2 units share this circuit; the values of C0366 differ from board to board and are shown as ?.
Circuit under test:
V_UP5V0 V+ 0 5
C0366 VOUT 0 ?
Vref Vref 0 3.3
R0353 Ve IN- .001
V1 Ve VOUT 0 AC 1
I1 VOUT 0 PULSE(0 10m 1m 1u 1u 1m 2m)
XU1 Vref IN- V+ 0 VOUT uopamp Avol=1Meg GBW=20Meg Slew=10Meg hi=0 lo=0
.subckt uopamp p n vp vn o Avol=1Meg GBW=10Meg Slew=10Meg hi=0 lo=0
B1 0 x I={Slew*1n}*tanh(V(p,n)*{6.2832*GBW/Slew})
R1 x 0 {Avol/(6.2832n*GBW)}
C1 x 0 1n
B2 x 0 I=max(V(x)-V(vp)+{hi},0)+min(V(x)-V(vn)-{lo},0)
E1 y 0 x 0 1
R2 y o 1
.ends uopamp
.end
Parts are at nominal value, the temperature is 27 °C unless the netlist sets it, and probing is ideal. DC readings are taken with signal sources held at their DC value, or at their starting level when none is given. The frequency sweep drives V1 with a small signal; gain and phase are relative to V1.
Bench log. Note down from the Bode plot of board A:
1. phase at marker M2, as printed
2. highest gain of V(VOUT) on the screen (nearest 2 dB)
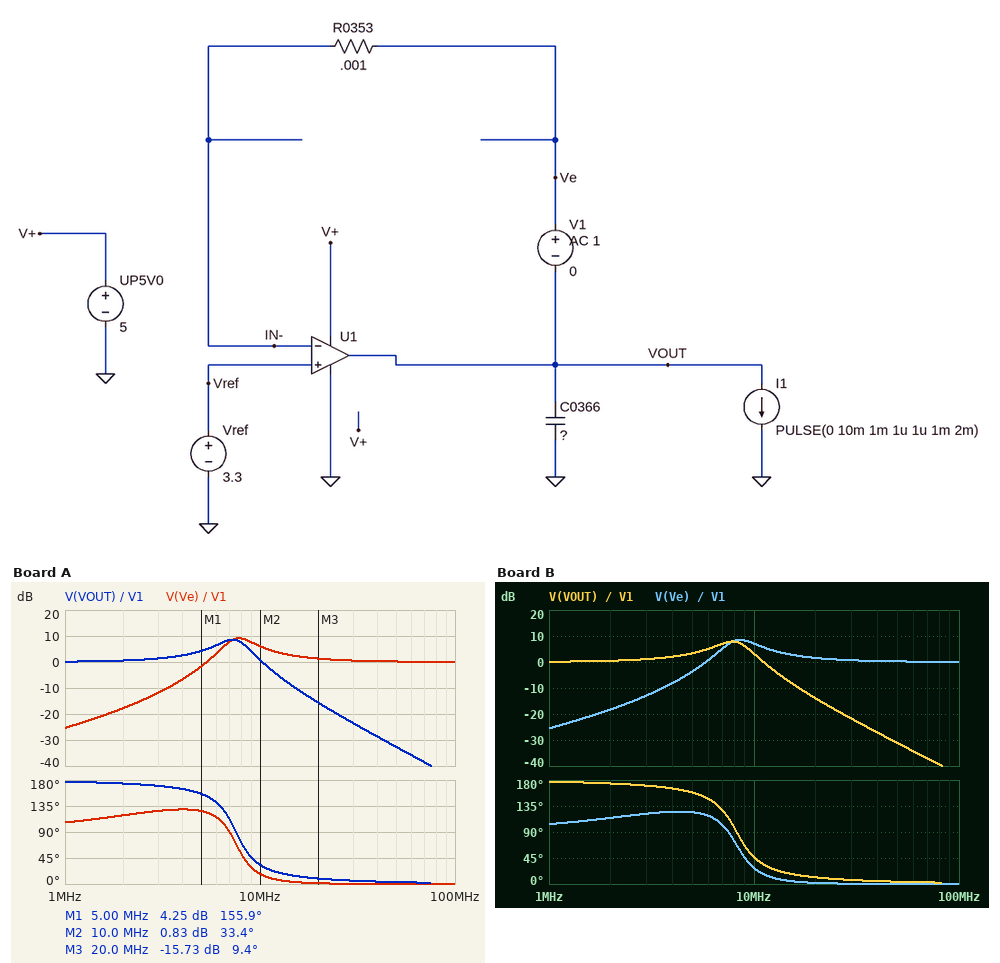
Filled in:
33.4 deg
8 dB
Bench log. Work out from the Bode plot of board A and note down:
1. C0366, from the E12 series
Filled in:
56 nF
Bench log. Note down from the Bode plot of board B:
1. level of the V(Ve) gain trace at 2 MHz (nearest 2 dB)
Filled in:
-18 dB
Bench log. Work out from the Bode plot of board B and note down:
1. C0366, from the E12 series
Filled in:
47 nF
